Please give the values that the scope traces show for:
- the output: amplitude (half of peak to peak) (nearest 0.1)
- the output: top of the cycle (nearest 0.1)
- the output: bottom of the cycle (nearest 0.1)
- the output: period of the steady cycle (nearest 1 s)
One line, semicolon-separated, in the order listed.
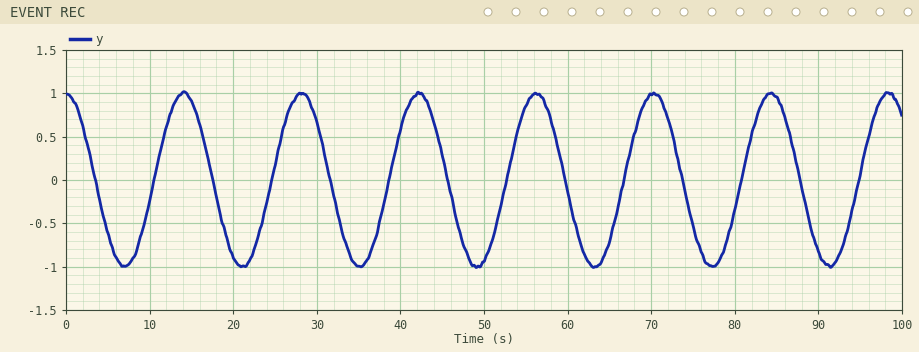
1.0; 1.0; -1.0; 14 s
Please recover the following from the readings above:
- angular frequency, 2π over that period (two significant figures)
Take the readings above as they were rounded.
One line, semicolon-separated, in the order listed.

0.45 rad/s
